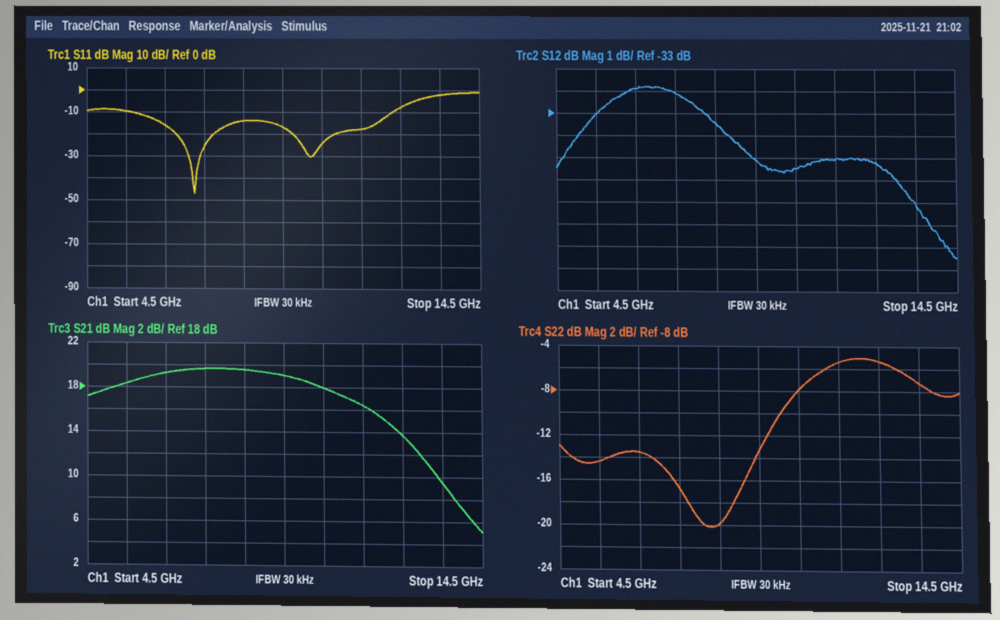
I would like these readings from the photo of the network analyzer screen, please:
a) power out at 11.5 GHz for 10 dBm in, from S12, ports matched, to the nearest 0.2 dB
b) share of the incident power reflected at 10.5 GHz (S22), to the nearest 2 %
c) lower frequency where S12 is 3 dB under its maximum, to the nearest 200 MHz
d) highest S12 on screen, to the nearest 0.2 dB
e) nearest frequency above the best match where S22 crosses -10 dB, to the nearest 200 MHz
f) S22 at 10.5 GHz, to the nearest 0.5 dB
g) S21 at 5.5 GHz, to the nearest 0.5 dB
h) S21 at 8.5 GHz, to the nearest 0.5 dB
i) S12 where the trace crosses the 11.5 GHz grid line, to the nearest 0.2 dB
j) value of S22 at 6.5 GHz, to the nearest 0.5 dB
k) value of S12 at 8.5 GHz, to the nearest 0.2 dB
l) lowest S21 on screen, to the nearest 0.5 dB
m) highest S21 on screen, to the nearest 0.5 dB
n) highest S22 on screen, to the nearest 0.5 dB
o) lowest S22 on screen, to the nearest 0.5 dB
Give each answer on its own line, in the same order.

-25.0 dBm
16 %
4.8 GHz
-31.8 dB
10.0 GHz
-8.0 dB
18.5 dB
19.5 dB
-35.0 dB
-13.5 dB
-33.4 dB
5.0 dB
19.5 dB
-5.0 dB
-20.0 dB
